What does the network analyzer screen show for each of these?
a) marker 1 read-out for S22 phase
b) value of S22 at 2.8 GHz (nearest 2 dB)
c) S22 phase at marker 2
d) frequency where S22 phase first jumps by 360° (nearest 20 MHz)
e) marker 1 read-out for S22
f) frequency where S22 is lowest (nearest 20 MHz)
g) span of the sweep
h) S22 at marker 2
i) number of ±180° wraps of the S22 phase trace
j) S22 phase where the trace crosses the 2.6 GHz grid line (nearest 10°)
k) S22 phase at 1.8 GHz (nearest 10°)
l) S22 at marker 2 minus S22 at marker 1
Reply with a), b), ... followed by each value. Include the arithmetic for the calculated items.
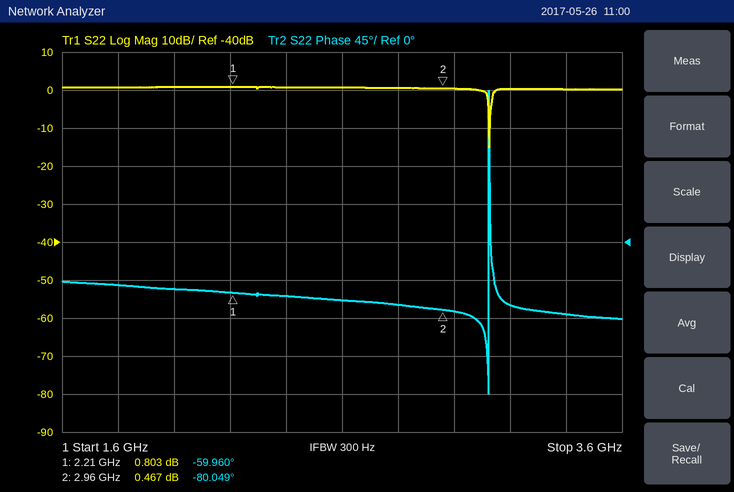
a) -59.960°
b) 0 dB
c) -80.049°
d) 3.12 GHz
e) 0.803 dB
f) 3.12 GHz
g) 2 GHz
h) 0.467 dB
i) 1
j) -70°
k) -50°
l) 0.467 − (0.803) = -0.336 dB
